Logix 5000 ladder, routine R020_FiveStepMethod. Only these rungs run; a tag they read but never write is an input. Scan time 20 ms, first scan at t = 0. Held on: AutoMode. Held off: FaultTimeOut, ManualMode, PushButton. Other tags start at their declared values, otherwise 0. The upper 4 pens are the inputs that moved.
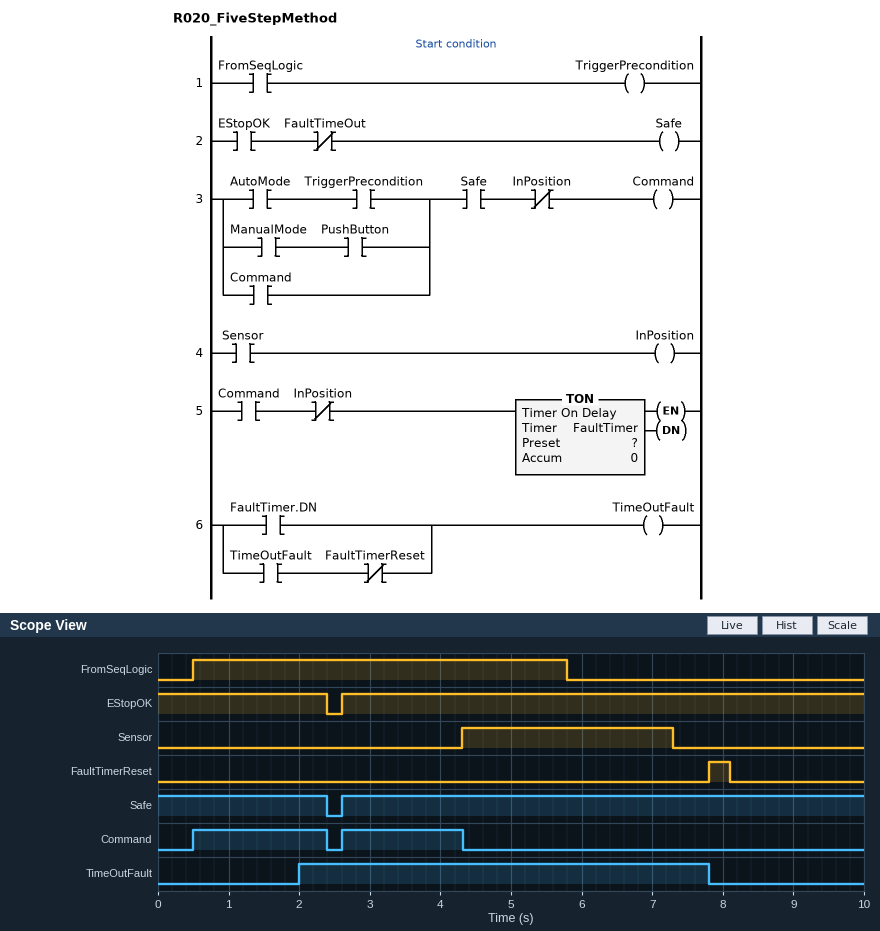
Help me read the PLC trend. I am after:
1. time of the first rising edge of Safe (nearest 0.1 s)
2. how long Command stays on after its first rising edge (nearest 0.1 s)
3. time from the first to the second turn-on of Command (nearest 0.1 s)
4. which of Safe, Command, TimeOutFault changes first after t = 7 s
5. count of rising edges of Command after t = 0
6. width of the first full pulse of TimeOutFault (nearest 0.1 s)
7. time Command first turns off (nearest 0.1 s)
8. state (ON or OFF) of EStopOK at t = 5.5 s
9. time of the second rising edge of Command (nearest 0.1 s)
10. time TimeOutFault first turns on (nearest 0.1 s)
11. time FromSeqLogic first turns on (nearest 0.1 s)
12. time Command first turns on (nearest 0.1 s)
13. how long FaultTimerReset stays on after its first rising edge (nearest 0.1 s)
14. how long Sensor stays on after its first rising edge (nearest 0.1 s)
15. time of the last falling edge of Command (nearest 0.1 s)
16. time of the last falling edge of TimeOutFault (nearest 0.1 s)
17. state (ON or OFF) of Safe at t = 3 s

2.6 s
1.9 s
2.1 s
TimeOutFault
2
5.8 s
2.4 s
ON
2.6 s
2.0 s
0.5 s
0.5 s
0.3 s
3.0 s
4.3 s
7.8 s
ON
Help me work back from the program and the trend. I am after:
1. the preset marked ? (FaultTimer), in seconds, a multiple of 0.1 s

1.5 s
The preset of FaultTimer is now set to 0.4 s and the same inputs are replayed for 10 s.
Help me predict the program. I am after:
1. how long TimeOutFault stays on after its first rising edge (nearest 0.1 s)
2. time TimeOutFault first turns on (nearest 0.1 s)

6.9 s
0.9 s
